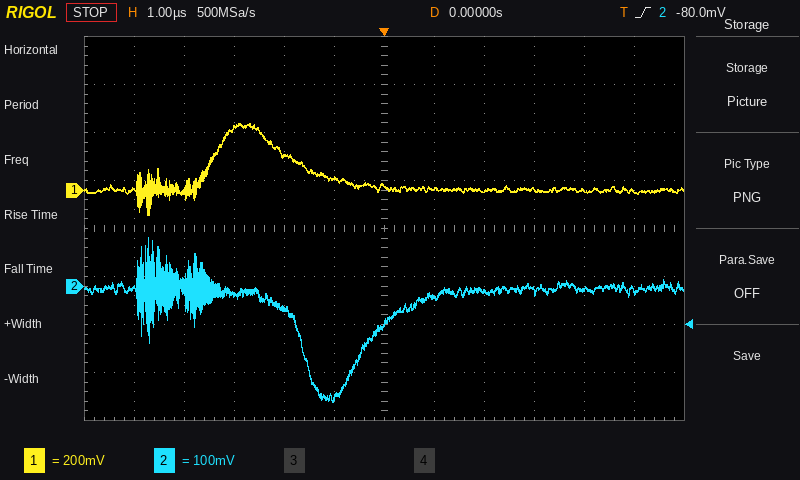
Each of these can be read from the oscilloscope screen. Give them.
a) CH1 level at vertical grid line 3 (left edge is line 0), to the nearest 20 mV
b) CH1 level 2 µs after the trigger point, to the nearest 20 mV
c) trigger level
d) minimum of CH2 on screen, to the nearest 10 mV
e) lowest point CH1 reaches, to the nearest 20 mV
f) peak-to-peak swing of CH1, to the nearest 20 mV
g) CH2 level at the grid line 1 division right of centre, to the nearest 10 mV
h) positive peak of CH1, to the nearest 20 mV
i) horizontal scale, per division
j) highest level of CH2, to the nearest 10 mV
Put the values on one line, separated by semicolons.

260 mV; 0 mV; -80.0 mV; -240 mV; -100 mV; 380 mV; -20 mV; 280 mV; 1 µs; 100 mV
